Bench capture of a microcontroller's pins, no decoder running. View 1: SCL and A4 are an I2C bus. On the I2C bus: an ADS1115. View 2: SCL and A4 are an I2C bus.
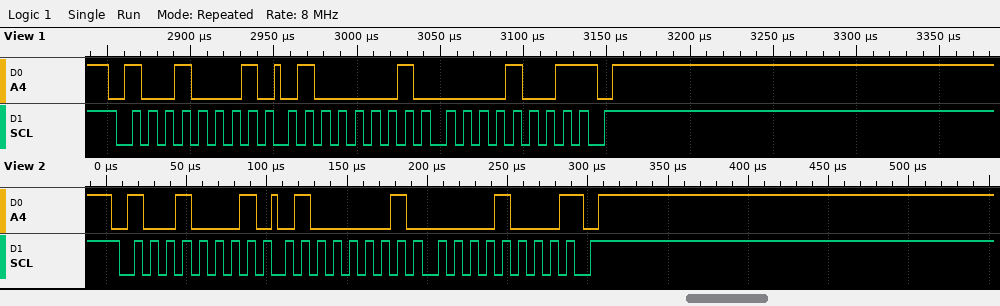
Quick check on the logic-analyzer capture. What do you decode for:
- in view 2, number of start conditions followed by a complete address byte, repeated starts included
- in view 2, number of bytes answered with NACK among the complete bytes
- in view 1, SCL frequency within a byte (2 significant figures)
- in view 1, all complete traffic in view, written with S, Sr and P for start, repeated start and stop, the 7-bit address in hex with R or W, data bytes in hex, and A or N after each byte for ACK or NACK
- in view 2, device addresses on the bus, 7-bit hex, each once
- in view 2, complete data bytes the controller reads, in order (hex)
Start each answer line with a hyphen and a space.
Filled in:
- 1
- 1
- 100 kHz
- S 48R A 41 A 09 N P
- 0x48
- 41 08
